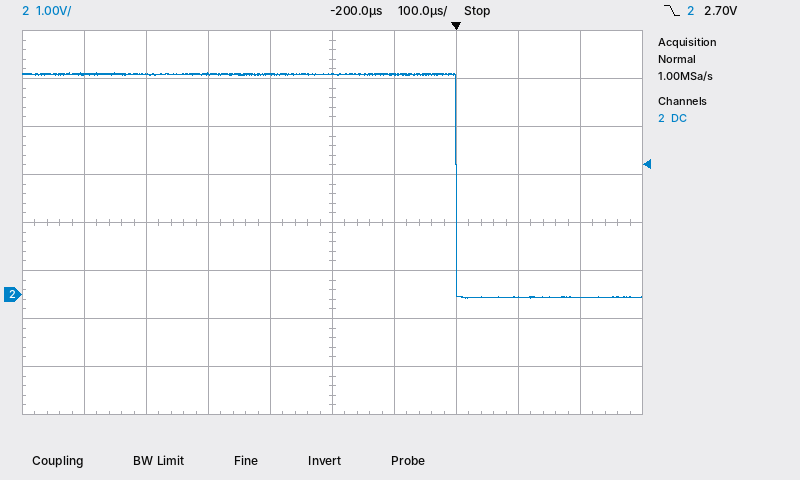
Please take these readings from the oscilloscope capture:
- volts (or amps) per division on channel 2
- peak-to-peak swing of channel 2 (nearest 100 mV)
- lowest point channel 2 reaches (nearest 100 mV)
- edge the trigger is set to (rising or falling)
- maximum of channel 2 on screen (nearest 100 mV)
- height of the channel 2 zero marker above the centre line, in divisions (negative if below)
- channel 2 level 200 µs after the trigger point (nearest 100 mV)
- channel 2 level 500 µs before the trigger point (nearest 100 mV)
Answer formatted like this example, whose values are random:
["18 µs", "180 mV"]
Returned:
["1 V", "4.7 V", "-100 mV", "falling", "4.6 V", "-1.5 div", "-100 mV", "4.6 V"]
